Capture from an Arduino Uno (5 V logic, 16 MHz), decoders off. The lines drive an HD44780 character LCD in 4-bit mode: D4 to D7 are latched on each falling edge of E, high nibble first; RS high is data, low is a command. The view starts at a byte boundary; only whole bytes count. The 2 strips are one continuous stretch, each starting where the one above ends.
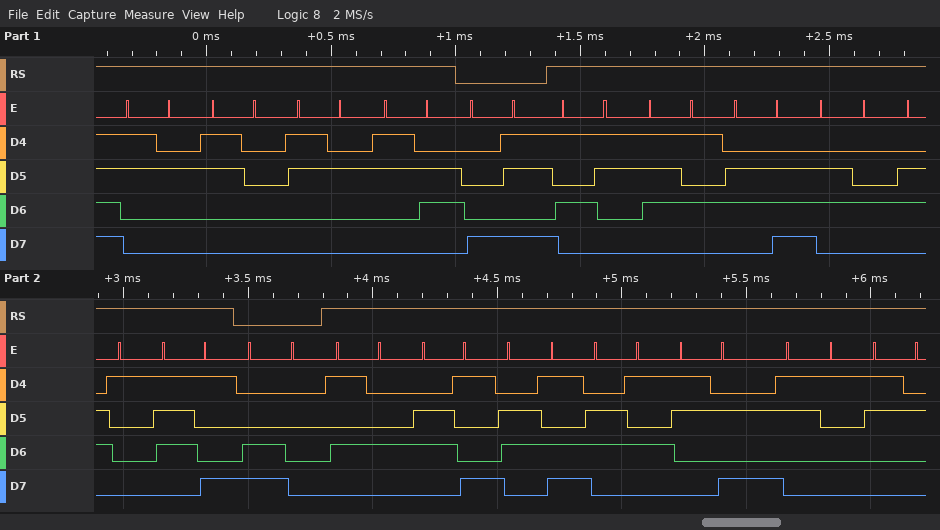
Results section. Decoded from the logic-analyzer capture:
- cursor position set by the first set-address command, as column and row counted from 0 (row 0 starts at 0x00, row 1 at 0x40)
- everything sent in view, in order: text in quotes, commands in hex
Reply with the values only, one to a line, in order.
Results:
column 11, row 0
"2026" 0x8B "Sunday" 0xC0 "Time:12"
